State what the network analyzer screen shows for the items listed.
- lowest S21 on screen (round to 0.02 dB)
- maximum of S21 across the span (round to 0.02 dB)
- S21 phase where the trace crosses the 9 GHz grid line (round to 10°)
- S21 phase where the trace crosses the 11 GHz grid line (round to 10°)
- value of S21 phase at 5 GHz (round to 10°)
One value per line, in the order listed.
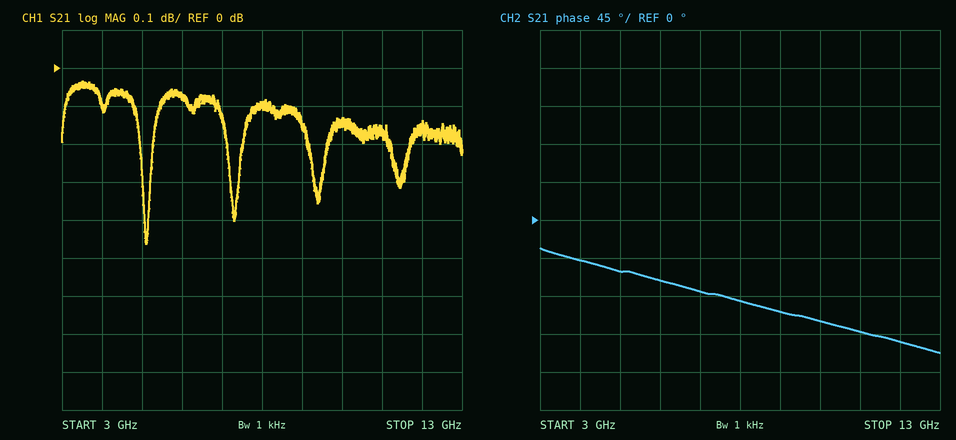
-0.46 dB
-0.04 dB
-110°
-130°
-60°
